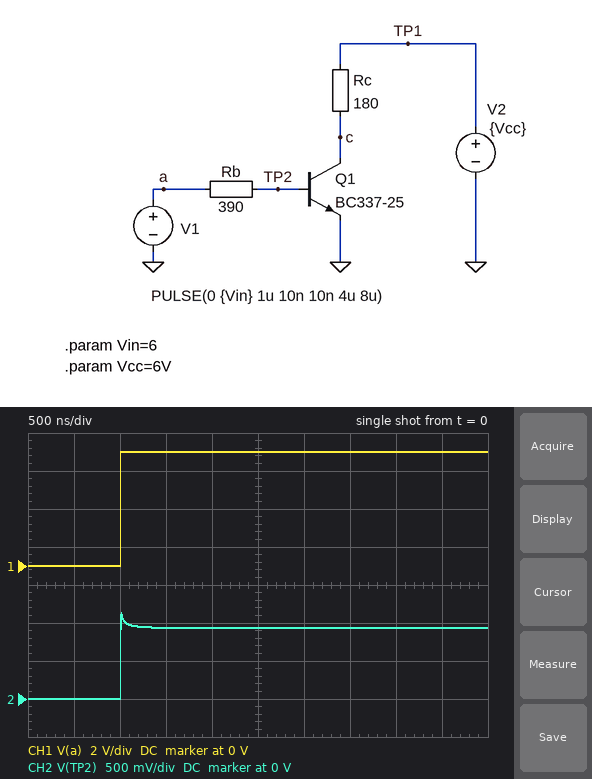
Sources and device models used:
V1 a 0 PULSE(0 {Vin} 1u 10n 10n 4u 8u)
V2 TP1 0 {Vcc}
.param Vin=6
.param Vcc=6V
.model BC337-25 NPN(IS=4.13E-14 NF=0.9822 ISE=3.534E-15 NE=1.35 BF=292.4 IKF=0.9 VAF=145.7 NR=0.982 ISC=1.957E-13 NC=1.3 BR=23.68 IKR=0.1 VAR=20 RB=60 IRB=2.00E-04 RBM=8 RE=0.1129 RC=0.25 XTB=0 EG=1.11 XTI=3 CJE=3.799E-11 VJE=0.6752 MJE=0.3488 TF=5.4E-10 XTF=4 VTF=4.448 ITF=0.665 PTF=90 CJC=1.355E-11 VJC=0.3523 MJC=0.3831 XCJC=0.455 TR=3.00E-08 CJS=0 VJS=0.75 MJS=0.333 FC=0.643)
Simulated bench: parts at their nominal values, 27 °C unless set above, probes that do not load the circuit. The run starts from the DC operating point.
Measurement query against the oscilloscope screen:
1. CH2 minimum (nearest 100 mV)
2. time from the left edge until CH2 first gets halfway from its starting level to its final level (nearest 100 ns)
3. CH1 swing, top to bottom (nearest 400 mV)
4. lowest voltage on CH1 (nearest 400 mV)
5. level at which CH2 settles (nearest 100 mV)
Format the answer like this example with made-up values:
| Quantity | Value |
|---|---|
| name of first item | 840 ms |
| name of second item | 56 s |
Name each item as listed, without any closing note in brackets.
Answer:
| Quantity | Value |
|---|---|
| CH2 minimum | 0 V |
| time from the left edge until CH2 first gets halfway from its starting level to its final level | 1.0 µs |
| CH1 swing, top to bottom | 6.0 V |
| lowest voltage on CH1 | 0 V |
| level at which CH2 settles | 900 mV |
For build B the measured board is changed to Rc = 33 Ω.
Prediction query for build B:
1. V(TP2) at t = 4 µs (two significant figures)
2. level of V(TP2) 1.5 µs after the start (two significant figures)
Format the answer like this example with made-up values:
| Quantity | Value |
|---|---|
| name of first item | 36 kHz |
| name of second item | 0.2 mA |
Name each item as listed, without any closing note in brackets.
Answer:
| Quantity | Value |
|---|---|
| V(TP2) at t = 4 µs | 960 mV |
| level of V(TP2) 1.5 µs after the start | 970 mV |
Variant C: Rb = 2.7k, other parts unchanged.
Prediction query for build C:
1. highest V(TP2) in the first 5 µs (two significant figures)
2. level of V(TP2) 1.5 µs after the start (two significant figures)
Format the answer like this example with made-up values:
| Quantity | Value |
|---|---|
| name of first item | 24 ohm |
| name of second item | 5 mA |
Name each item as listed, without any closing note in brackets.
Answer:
| Quantity | Value |
|---|---|
| highest V(TP2) in the first 5 µs | 770 mV |
| level of V(TP2) 1.5 µs after the start | 760 mV |
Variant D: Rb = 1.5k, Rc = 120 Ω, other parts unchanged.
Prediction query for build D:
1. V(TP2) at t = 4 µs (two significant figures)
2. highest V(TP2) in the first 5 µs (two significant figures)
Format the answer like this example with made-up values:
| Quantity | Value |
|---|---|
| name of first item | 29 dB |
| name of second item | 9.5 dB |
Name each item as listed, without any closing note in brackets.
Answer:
| Quantity | Value |
|---|---|
| V(TP2) at t = 4 µs | 800 mV |
| highest V(TP2) in the first 5 µs | 830 mV |
